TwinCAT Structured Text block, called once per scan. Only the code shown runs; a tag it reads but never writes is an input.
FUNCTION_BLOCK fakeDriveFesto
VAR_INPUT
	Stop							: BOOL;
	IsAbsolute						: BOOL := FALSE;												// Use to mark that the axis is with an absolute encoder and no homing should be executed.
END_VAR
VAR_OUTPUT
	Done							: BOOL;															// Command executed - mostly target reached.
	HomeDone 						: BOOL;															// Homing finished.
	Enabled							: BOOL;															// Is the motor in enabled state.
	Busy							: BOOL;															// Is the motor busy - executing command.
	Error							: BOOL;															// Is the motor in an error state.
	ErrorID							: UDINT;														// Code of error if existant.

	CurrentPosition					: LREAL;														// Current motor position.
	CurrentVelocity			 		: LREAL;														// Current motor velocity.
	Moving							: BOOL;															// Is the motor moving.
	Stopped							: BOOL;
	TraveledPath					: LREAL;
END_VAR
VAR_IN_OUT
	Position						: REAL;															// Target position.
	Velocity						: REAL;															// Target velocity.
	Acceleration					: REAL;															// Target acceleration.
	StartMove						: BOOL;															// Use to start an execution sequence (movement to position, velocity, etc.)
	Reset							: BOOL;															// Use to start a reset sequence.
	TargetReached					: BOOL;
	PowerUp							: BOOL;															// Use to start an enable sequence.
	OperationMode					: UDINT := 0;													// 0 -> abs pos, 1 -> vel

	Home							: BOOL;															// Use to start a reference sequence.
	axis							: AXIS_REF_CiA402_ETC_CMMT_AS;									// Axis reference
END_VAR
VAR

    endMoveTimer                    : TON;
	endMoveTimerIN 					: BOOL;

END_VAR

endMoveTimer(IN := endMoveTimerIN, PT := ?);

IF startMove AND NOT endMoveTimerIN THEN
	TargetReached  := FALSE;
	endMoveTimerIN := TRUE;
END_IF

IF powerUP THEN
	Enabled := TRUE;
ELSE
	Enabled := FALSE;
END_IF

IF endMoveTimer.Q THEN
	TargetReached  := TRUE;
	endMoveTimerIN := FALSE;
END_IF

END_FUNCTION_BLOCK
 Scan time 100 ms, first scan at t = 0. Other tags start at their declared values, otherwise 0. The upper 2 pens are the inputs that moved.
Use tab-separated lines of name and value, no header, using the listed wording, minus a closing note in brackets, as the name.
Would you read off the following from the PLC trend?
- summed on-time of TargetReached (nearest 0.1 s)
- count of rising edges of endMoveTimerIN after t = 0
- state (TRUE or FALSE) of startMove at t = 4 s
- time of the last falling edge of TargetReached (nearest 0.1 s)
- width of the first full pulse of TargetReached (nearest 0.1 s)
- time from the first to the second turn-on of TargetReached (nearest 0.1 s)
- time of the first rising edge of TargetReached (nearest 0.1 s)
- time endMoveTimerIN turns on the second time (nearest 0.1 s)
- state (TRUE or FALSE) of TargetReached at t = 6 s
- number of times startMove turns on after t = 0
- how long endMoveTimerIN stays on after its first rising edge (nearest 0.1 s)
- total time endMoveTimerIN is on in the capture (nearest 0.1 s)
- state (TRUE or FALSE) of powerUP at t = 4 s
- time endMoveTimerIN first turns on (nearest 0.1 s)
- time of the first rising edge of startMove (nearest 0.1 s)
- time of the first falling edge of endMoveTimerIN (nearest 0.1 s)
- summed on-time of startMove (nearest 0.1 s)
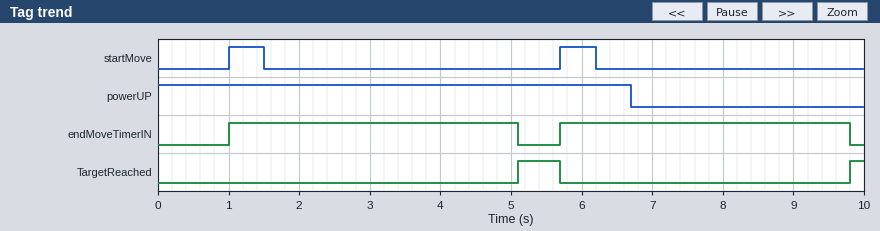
summed on-time of TargetReached	0.8 s
count of rising edges of endMoveTimerIN after t = 0	2
state (TRUE or FALSE) of startMove at t = 4 s	FALSE
time of the last falling edge of TargetReached	5.7 s
width of the first full pulse of TargetReached	0.6 s
time from the first to the second turn-on of TargetReached	4.7 s
time of the first rising edge of TargetReached	5.1 s
time endMoveTimerIN turns on the second time	5.7 s
state (TRUE or FALSE) of TargetReached at t = 6 s	FALSE
number of times startMove turns on after t = 0	2
how long endMoveTimerIN stays on after its first rising edge	4.1 s
total time endMoveTimerIN is on in the capture	8.2 s
state (TRUE or FALSE) of powerUP at t = 4 s	TRUE
time endMoveTimerIN first turns on	1.0 s
time of the first rising edge of startMove	1.0 s
time of the first falling edge of endMoveTimerIN	5.1 s
summed on-time of startMove	1.0 s
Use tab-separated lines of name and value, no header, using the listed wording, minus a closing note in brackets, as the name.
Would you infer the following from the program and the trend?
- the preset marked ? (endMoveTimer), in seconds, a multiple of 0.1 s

the preset marked ? (endMoveTimer), in seconds, a multiple of 0.1 s	4.0 s
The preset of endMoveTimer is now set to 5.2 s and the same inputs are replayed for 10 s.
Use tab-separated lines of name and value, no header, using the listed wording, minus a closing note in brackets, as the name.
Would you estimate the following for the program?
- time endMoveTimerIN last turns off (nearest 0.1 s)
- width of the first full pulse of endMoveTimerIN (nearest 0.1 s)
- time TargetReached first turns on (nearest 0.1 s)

time endMoveTimerIN last turns off	6.3 s
width of the first full pulse of endMoveTimerIN	5.3 s
time TargetReached first turns on	6.3 s
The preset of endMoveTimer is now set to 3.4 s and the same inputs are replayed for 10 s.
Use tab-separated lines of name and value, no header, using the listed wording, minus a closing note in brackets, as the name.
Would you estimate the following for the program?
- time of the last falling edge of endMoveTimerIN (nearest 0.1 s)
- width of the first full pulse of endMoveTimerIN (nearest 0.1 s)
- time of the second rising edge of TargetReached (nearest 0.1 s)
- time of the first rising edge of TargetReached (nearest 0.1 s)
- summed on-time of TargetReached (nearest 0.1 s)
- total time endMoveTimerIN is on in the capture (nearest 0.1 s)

time of the last falling edge of endMoveTimerIN	9.2 s
width of the first full pulse of endMoveTimerIN	3.5 s
time of the second rising edge of TargetReached	9.2 s
time of the first rising edge of TargetReached	4.5 s
summed on-time of TargetReached	2.0 s
total time endMoveTimerIN is on in the capture	7.0 s
